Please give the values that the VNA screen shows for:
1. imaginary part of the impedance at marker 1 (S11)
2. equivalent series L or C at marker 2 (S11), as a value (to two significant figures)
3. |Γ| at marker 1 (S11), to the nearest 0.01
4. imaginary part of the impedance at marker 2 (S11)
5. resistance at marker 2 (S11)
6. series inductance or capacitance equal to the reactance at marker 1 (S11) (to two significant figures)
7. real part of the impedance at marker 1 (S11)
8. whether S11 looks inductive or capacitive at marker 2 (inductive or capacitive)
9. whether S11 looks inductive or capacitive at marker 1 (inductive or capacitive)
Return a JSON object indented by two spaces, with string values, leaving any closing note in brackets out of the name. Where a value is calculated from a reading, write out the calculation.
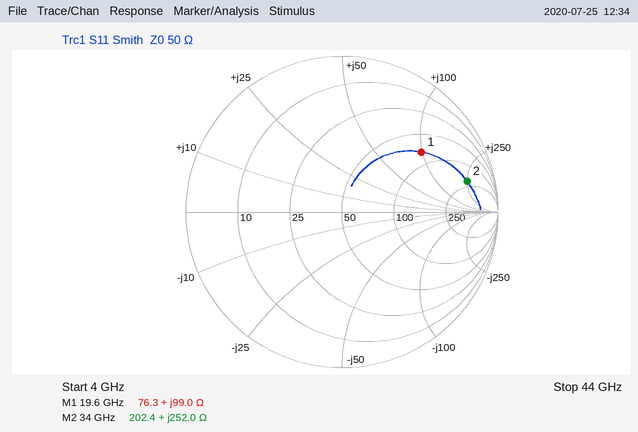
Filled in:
{
  "imaginary part of the impedance at marker 1": "+99.0 Ω",
  "equivalent series L or C at marker 2 (S11), as a value": "L = 252 Ω/(2π × 34 GHz) ≈ 1.2 nH",
  "|Γ| at marker 1 (S11), to the nearest 0.01": "0.64",
  "imaginary part of the impedance at marker 2": "+252.0 Ω",
  "resistance at marker 2": "202.4 Ω",
  "series inductance or capacitance equal to the reactance at marker 1 (S11)": "L = 99 Ω/(2π × 19.6 GHz) ≈ 804 pH, so 800 pH to two significant figures",
  "real part of the impedance at marker 1": "76.3 Ω",
  "whether S11 looks inductive or capacitive at marker 2": "inductive",
  "whether S11 looks inductive or capacitive at marker 1": "inductive"
}
